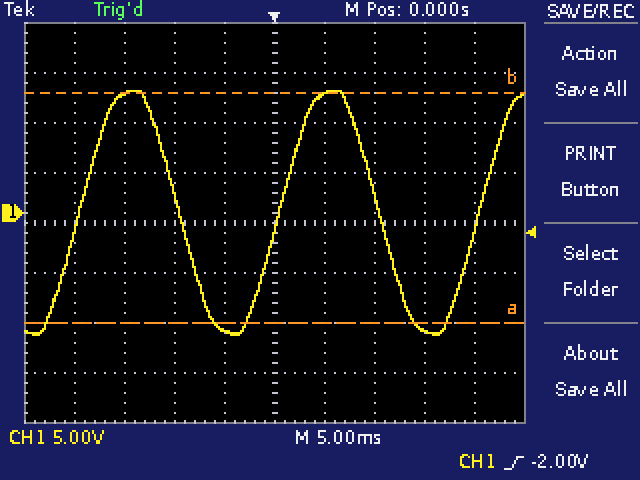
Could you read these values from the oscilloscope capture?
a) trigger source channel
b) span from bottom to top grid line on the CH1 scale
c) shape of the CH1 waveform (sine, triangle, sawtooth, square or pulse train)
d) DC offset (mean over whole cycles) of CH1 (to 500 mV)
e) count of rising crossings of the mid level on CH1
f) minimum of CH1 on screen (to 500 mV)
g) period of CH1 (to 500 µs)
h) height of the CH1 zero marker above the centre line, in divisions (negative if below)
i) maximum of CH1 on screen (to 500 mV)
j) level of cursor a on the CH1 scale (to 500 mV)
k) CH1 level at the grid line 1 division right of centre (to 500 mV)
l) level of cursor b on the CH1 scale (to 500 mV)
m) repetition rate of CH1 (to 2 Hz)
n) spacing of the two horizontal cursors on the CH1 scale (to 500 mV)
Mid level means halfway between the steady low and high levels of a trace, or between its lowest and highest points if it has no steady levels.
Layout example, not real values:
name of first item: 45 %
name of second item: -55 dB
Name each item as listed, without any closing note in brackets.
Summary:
trigger source channel: CH1
span from bottom to top grid line on the CH1 scale: 40 V
shape of the CH1 waveform: sine
DC offset (mean over whole cycles) of CH1: 0.0 V
count of rising crossings of the mid level on CH1: 3
minimum of CH1 on screen: -12.0 V
period of CH1: 20.0 ms
height of the CH1 zero marker above the centre line, in divisions: +0.2 div
maximum of CH1 on screen: 12.0 V
level of cursor a on the CH1 scale: -11.0 V
CH1 level at the grid line 1 division right of centre: 12.0 V
level of cursor b on the CH1 scale: 12.0 V
repetition rate of CH1: 50 Hz
spacing of the two horizontal cursors on the CH1 scale: 23.0 V
